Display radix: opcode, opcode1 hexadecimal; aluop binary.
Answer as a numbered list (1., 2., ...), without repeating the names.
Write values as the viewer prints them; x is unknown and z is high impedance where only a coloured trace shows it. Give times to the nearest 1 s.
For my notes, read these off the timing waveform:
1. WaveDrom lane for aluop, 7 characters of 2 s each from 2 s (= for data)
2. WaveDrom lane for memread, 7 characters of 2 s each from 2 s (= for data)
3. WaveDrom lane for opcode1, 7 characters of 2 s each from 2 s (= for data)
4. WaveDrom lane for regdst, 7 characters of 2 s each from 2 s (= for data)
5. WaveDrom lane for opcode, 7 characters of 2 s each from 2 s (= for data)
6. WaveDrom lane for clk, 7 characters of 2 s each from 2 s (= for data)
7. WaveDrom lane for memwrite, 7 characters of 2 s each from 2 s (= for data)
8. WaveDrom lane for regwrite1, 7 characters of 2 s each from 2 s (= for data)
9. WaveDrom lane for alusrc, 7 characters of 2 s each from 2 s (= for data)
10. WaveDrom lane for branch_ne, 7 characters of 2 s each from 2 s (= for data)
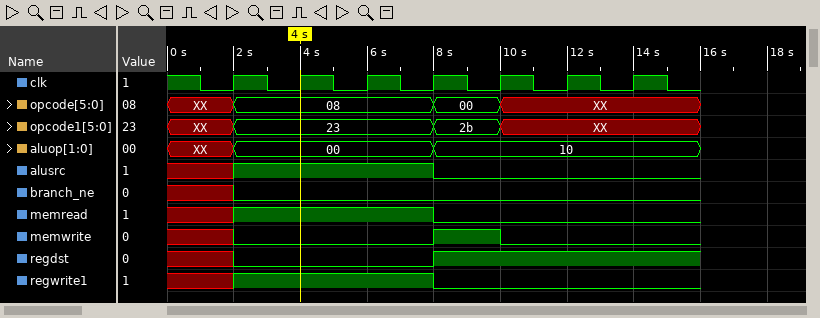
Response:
1. {name: 'aluop', wave: '=..=...', data: '00 10'}
2. {name: 'memread', wave: '1..0...'}
3. {name: 'opcode1', wave: '=..=x..', data: '23 2b'}
4. {name: 'regdst', wave: '0..1...'}
5. {name: 'opcode', wave: '=..=x..', data: '08 00'}
6. {name: 'clk', wave: 'p......'}
7. {name: 'memwrite', wave: '0..10..'}
8. {name: 'regwrite1', wave: '1..0...'}
9. {name: 'alusrc', wave: '1..0...'}
10. {name: 'branch_ne', wave: '0......'}
